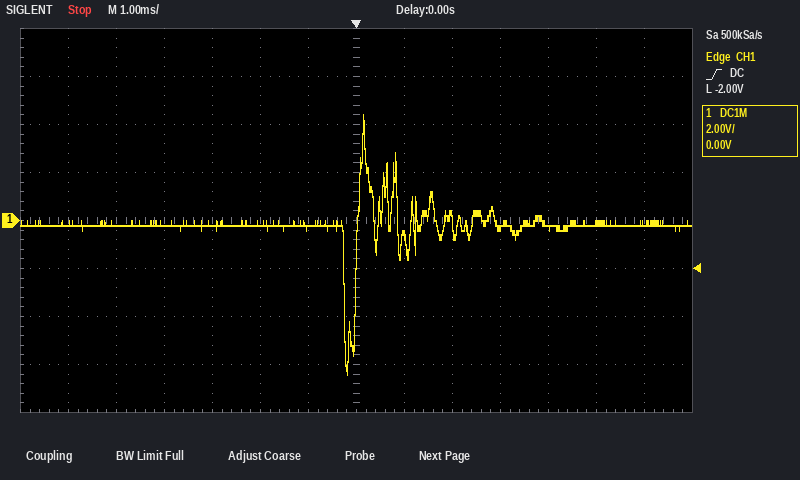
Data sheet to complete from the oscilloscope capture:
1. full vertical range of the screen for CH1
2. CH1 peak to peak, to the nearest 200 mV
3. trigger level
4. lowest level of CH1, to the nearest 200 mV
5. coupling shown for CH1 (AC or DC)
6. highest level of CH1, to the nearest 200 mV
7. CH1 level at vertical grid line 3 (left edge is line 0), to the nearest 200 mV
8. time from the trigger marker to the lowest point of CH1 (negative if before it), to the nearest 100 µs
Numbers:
16 V
10.8 V
-2.00 V
-6.4 V
DC
4.4 V
-200 mV
-200 µs
